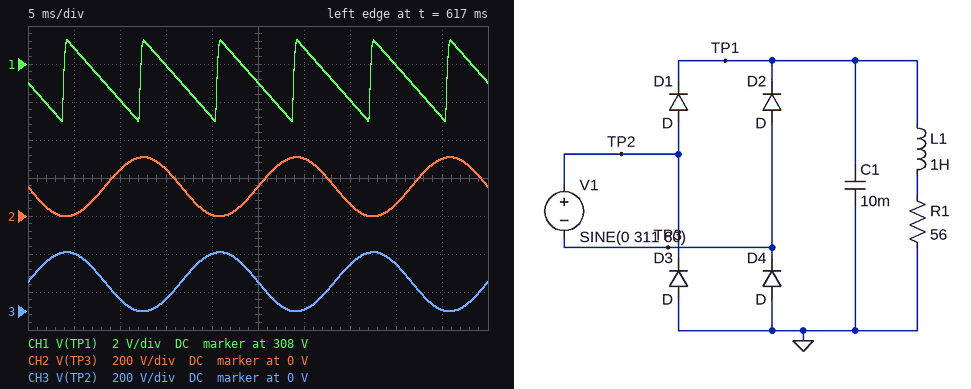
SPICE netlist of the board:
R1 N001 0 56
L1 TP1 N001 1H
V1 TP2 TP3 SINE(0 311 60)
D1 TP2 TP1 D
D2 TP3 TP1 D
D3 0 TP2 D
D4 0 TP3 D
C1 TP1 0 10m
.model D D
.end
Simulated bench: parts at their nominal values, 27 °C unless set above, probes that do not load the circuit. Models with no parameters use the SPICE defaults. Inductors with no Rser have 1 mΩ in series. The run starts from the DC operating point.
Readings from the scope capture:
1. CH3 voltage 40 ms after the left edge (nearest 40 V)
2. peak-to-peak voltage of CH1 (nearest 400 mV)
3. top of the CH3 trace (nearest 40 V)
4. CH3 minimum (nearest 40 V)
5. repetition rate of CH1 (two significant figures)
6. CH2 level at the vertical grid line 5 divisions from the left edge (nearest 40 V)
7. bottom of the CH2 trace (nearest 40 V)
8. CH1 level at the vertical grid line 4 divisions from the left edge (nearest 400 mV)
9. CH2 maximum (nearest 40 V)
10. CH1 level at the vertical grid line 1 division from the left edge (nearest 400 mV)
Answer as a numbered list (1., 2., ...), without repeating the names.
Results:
1. 240 V
2. 4.4 V
3. 320 V
4. 0 V
5. 120 Hz
6. 160 V
7. 0 V
8. 305.2 V
9. 320 V
10. 308.8 V
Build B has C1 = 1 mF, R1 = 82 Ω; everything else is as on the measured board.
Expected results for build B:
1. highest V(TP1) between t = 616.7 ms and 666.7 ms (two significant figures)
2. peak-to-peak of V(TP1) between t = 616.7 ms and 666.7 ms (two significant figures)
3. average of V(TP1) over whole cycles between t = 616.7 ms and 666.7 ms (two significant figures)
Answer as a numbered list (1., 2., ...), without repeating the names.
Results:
1. 310 V
2. 26 V
3. 300 V
